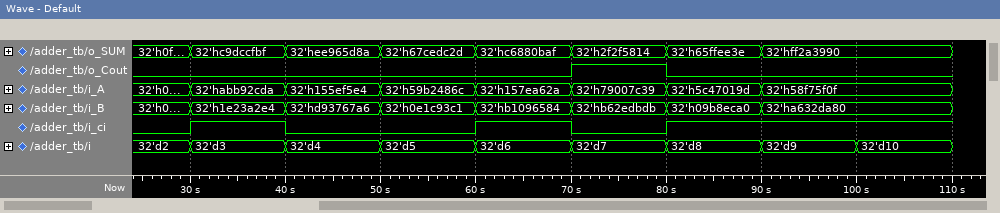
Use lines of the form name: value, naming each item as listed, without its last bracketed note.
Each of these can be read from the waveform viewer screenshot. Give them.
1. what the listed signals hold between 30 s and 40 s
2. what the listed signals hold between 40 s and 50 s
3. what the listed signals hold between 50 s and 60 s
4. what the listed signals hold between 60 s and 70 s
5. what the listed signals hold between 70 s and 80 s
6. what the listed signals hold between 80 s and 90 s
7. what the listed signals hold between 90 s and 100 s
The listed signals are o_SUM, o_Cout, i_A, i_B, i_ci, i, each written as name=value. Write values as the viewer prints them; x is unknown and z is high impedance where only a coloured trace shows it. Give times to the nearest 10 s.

what the listed signals hold between 30 s and 40 s: o_SUM=32'hc9dccfbf, o_Cout=0, i_A=32'habb92cda, i_B=32'h1e23a2e4, i_ci=1, i=32'd3
what the listed signals hold between 40 s and 50 s: o_SUM=32'hee965d8a, o_Cout=0, i_A=32'h155ef5e4, i_B=32'hd93767a6, i_ci=0, i=32'd4
what the listed signals hold between 50 s and 60 s: o_SUM=32'h67cedc2d, o_Cout=0, i_A=32'h59b2486c, i_B=32'h0e1c93c1, i_ci=0, i=32'd5
what the listed signals hold between 60 s and 70 s: o_SUM=32'hc6880baf, o_Cout=0, i_A=32'h157ea62a, i_B=32'hb1096584, i_ci=1, i=32'd6
what the listed signals hold between 70 s and 80 s: o_SUM=32'h2f2f5814, o_Cout=1, i_A=32'h79007c39, i_B=32'hb62edbdb, i_ci=0, i=32'd7
what the listed signals hold between 80 s and 90 s: o_SUM=32'h65ffee3e, o_Cout=0, i_A=32'h5c47019d, i_B=32'h09b8eca0, i_ci=1, i=32'd8
what the listed signals hold between 90 s and 100 s: o_SUM=32'hff2a3990, o_Cout=0, i_A=32'h58f75f0f, i_B=32'ha632da80, i_ci=1, i=32'd9
